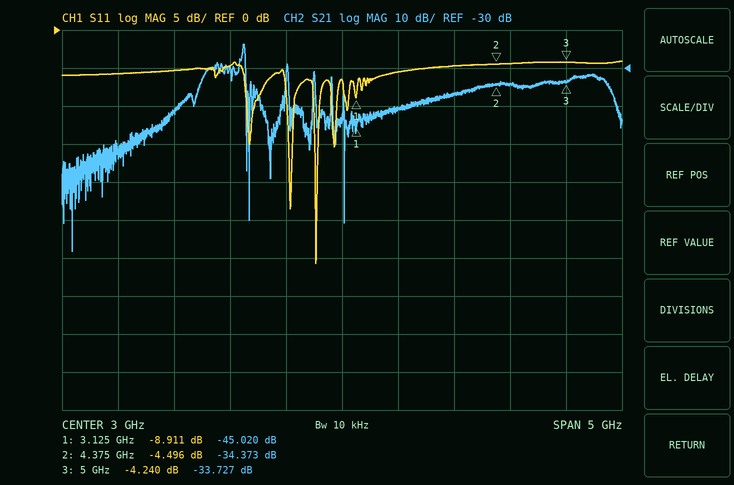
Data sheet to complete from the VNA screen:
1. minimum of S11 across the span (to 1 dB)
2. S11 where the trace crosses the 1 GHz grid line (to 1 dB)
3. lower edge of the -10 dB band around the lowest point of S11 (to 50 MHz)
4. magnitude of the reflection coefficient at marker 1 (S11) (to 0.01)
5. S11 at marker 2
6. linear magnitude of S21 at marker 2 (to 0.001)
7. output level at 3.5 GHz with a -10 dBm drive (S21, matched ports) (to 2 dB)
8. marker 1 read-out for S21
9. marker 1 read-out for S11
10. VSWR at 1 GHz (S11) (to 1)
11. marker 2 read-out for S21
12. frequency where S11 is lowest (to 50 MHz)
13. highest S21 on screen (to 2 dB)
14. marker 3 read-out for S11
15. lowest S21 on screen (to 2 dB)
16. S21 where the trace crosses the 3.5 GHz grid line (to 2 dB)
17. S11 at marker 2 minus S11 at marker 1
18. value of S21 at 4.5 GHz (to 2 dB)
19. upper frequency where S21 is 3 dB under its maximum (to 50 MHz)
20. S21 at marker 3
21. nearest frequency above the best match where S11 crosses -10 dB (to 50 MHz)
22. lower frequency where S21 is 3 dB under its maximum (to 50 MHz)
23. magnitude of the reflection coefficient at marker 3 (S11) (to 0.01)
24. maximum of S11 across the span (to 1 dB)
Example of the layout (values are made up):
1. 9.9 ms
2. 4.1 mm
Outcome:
1. -31 dB
2. -6 dB
3. 2.75 GHz
4. 0.36
5. -4.496 dB
6. 0.019
7. -50 dBm
8. -45.020 dB
9. -8.911 dB
10. 3
11. -34.373 dB
12. 2.75 GHz
13. -24 dB
14. -4.240 dB
15. -78 dB
16. -40 dB
17. 4.415 dB
18. -34 dB
19. 2.15 GHz
20. -33.727 dB
21. 2.80 GHz
22. 2.10 GHz
23. 0.61
24. -4 dB
